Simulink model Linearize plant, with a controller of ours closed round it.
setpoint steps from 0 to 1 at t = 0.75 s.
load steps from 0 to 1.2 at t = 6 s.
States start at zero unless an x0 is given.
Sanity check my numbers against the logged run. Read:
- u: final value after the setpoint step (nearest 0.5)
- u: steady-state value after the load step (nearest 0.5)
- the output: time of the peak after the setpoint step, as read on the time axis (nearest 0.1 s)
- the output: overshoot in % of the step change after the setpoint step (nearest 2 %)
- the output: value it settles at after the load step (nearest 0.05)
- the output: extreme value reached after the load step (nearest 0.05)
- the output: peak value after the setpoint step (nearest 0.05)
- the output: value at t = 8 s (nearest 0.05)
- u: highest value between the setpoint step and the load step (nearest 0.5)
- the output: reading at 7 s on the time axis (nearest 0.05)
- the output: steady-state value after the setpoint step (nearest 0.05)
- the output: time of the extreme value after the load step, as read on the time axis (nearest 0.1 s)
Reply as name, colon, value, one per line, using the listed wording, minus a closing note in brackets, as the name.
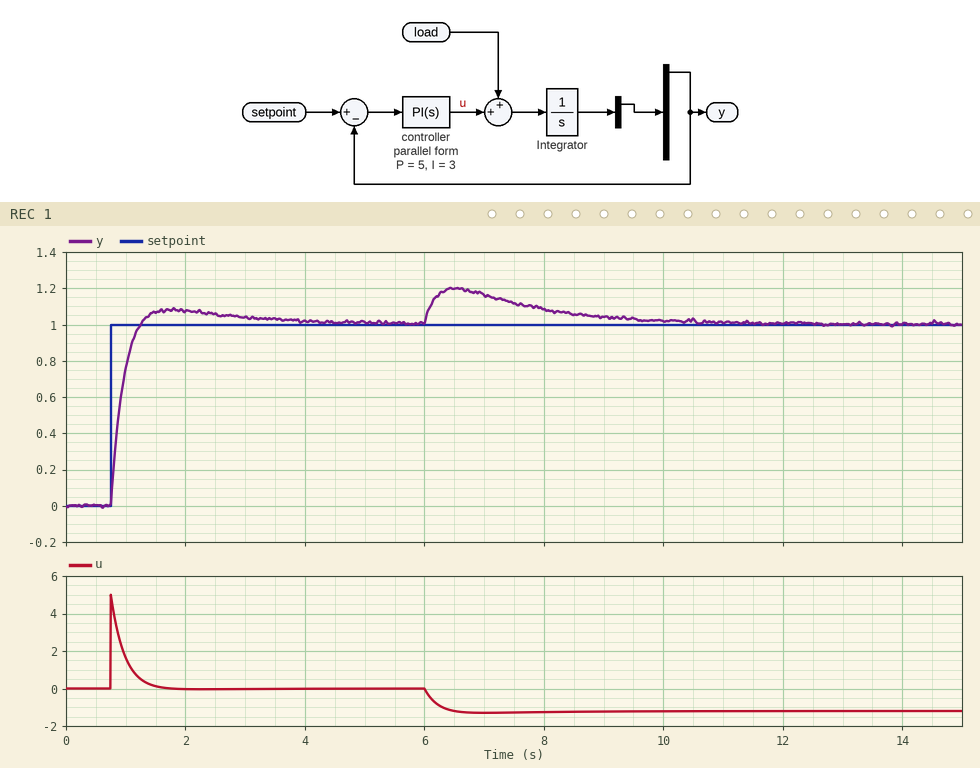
u: final value after the setpoint step: 0.0
u: steady-state value after the load step: -1.0
the output: time of the peak after the setpoint step, as read on the time axis: 1.8 s
the output: overshoot in % of the step change after the setpoint step: 8 %
the output: value it settles at after the load step: 1.00
the output: extreme value reached after the load step: 1.20
the output: peak value after the setpoint step: 1.10
the output: value at t = 8 s: 1.10
u: highest value between the setpoint step and the load step: 5.0
the output: reading at 7 s on the time axis: 1.15
the output: steady-state value after the setpoint step: 1.00
the output: time of the extreme value after the load step, as read on the time axis: 6.5 s
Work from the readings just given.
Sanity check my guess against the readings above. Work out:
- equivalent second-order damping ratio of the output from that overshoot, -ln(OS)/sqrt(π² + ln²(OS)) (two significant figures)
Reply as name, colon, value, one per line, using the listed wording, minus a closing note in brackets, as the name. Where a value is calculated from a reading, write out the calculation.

equivalent second-order damping ratio of the output from that overshoot, -ln(OS)/sqrt(π² + ln²(OS)): ln(0.08) = -2.526; 2.526 / sqrt(9.870 + 6.379) = 0.63
